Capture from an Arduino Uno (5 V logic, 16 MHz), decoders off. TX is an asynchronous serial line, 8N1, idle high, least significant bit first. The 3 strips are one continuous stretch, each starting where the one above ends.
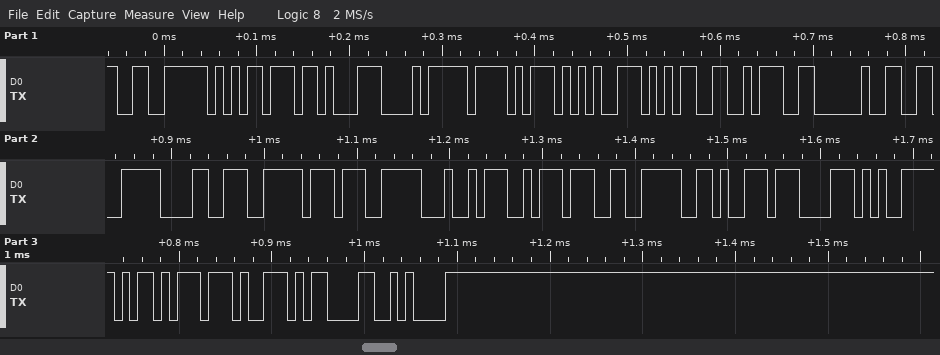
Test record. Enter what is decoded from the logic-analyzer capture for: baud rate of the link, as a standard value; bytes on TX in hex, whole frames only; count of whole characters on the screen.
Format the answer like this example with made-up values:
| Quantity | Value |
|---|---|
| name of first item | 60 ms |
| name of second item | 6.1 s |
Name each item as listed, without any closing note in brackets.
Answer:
| Quantity | Value |
|---|---|
| baud rate of the link, as a standard value | 115200 baud |
| bytes on TX in hex, whole frames only | 0xE6 0xB5 0x8B 0xE8 0xAF 0x95 0x35 0x3A 0x20 0xE6 0x98 0xBE 0xE7 0xA4 0xBA 0xE6 0x96 0x87 0xE5 0xAD 0x97 0x0D 0x0A |
| count of whole characters on the screen | 23 |
